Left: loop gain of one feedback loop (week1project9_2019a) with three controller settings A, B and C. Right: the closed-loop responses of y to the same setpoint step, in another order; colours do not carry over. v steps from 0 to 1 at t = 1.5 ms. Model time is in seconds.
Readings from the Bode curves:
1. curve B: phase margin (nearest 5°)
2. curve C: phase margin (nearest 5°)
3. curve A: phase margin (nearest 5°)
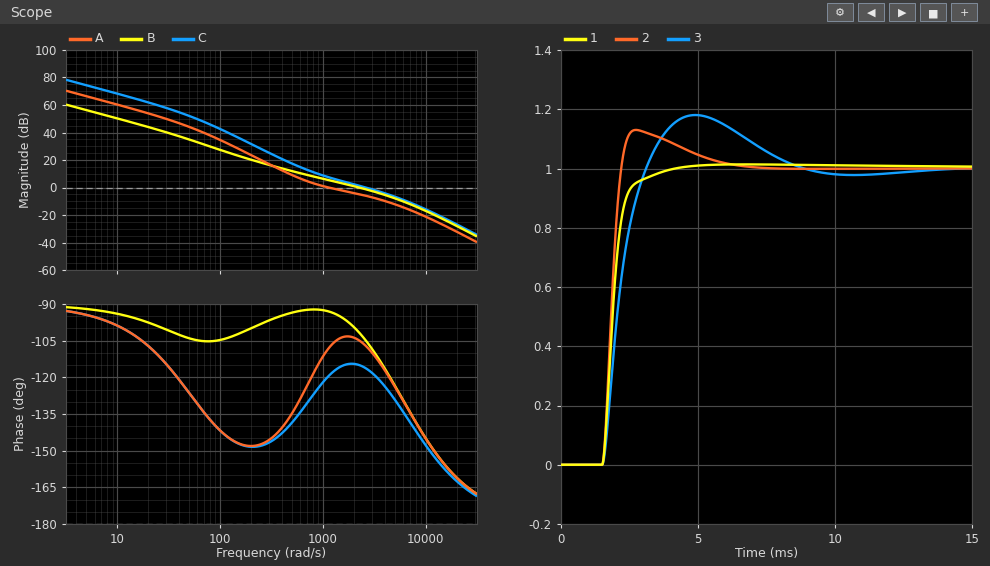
80°
65°
70°
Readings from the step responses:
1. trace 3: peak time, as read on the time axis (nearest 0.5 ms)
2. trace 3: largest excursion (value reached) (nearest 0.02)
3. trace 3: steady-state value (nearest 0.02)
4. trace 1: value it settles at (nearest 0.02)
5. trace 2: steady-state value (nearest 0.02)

5.0 ms
1.18
1.00
1.00
1.00
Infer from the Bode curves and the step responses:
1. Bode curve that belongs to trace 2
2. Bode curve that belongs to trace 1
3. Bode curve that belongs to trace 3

C
B
A
